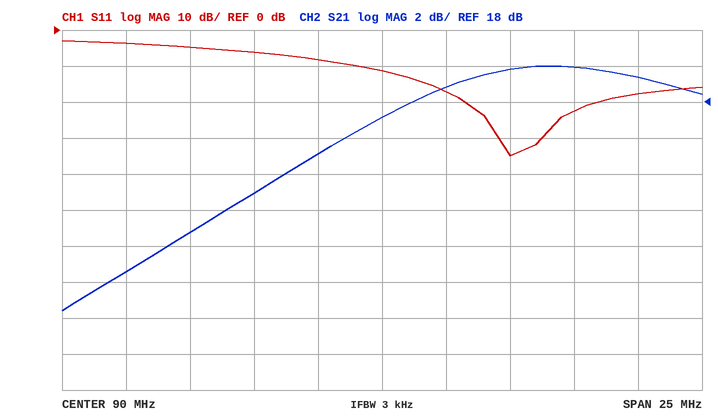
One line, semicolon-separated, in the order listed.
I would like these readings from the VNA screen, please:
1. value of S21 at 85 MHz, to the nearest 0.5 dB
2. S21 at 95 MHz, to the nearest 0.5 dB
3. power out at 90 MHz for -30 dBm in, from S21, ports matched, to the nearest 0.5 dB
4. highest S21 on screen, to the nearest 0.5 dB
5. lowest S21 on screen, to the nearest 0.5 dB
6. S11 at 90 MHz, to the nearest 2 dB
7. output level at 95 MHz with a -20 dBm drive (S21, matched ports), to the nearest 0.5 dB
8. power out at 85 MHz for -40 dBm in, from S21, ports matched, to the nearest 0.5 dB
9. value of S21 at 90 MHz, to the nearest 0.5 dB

13.0 dB; 20.0 dB; -13.0 dBm; 20.0 dB; 6.5 dB; -12 dB; 0.0 dBm; -27.0 dBm; 17.0 dB
